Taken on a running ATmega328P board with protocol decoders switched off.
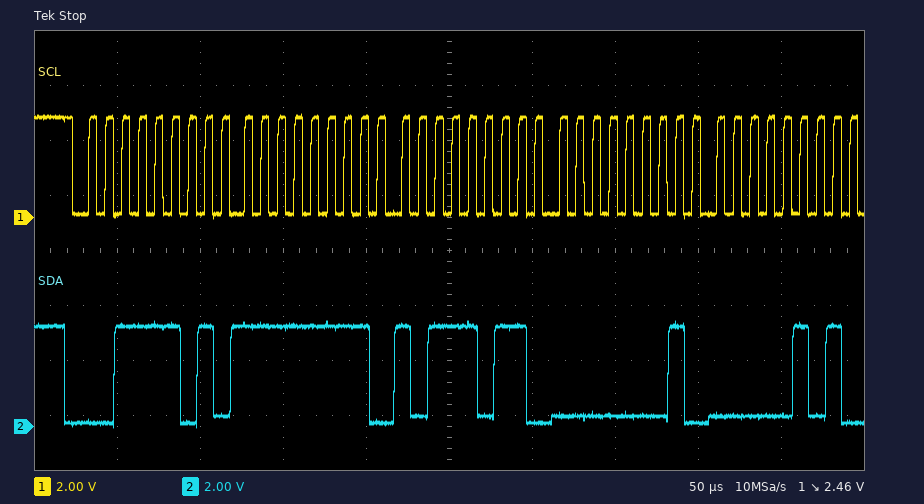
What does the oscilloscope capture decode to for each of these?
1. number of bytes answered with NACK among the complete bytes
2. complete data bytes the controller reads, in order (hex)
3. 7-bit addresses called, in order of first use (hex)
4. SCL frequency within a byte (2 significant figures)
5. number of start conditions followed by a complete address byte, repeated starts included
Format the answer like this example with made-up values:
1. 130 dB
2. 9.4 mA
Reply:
1. 0
2. FF BB 01 05
3. 0x1E
4. 100 kHz
5. 1
